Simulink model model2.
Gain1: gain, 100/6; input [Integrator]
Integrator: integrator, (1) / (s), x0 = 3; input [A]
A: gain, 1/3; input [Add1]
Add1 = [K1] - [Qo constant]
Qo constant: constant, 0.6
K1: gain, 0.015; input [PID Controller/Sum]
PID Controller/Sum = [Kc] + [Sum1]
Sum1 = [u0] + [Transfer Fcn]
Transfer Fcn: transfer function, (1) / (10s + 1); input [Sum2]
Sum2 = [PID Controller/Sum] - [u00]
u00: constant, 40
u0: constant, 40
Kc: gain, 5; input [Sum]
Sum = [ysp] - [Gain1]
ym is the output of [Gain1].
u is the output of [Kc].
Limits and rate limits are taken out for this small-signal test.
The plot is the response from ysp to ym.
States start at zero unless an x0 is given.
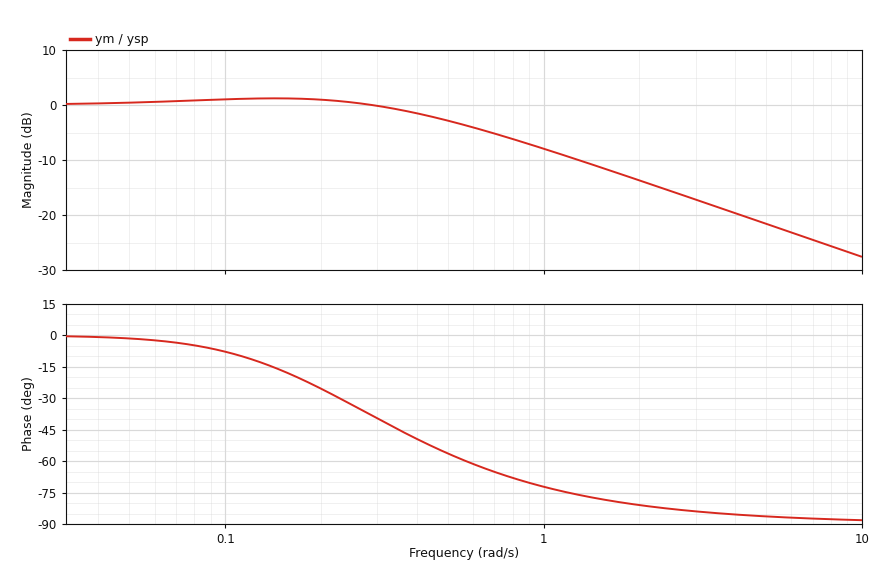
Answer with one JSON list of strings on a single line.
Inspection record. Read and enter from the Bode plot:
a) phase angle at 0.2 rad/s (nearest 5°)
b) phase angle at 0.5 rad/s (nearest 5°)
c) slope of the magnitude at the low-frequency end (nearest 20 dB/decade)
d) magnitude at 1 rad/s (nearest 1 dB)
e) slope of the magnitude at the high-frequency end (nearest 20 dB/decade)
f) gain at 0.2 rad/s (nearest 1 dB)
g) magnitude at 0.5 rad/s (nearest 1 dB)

["-25°", "-55°", "0 dB/decade", "-8 dB", "-20 dB/decade", "1 dB", "-3 dB"]
